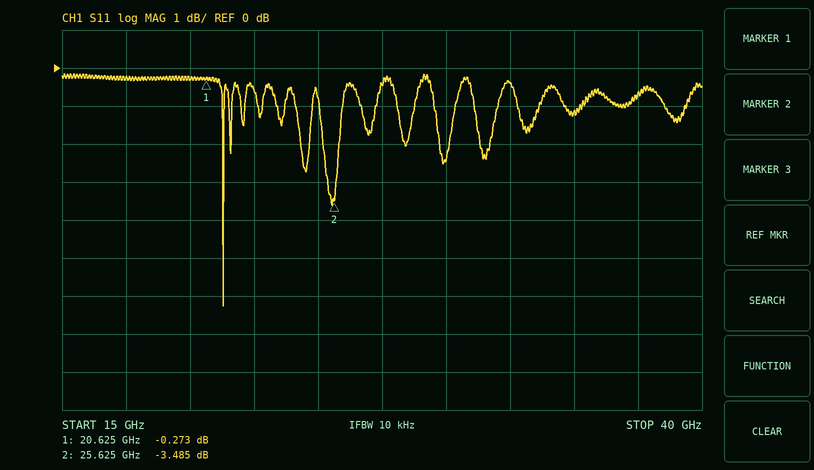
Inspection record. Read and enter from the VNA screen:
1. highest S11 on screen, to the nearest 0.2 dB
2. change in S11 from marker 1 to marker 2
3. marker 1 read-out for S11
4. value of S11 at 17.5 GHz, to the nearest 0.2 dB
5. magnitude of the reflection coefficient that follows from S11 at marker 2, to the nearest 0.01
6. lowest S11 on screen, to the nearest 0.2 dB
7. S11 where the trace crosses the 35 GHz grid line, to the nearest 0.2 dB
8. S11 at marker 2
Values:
-0.2 dB
-3.212 dB
-0.273 dB
-0.2 dB
0.67
-6.2 dB
-1.2 dB
-3.485 dB
